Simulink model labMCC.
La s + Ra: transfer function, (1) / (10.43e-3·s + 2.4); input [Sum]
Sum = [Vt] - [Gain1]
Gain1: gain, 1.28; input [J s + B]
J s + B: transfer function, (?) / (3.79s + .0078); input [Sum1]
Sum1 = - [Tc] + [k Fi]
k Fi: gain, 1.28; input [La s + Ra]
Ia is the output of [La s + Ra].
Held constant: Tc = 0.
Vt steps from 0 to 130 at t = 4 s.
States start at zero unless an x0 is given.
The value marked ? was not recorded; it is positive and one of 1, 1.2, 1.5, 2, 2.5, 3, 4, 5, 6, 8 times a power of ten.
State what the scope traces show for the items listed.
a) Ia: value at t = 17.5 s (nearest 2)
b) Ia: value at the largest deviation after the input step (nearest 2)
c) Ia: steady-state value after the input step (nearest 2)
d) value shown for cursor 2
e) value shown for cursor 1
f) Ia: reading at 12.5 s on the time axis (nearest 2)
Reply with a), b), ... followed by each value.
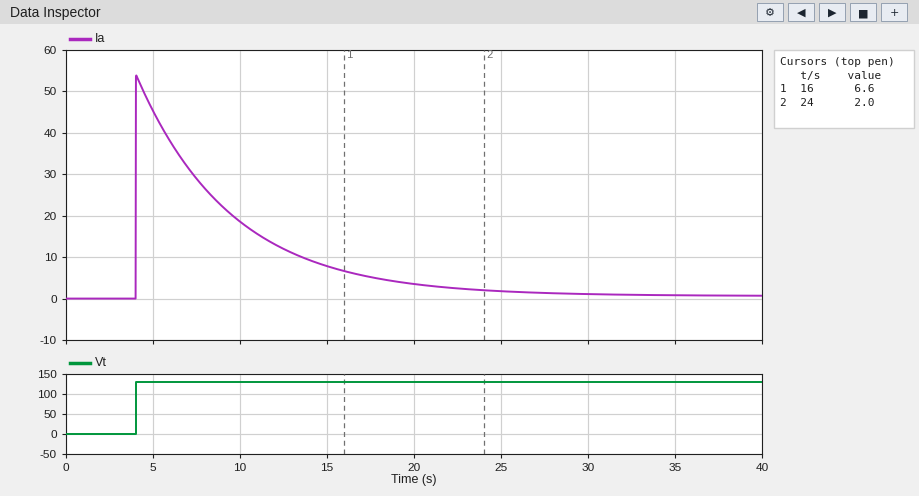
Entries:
a) 6
b) 54
c) 0
d) 2.0
e) 6.6
f) 12
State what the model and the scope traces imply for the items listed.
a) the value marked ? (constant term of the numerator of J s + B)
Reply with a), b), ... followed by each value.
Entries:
a) 1
